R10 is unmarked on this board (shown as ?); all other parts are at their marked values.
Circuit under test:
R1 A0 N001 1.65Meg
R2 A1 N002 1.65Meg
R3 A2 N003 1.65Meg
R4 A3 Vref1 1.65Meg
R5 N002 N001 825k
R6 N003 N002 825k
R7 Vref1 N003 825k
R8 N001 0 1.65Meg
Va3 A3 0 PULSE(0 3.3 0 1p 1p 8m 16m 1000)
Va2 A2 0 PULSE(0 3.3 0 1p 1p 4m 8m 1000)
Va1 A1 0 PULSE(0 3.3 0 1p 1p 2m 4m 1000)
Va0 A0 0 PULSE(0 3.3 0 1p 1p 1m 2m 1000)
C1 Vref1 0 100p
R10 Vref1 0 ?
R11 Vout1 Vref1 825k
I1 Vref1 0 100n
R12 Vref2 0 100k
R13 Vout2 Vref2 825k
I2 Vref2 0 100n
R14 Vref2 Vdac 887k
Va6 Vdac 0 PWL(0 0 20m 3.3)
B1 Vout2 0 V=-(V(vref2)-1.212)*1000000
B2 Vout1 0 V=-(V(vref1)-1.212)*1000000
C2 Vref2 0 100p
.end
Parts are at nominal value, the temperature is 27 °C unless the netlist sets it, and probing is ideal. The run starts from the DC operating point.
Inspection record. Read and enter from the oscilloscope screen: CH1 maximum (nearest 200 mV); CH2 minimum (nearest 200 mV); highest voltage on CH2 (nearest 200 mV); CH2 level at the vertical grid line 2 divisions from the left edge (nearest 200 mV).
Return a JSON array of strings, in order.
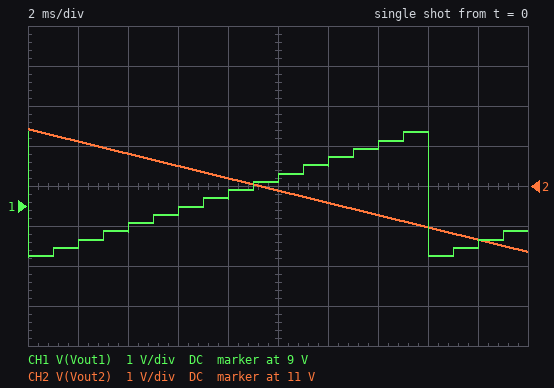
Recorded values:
["10.8 V", "9.4 V", "12.4 V", "11.8 V"]
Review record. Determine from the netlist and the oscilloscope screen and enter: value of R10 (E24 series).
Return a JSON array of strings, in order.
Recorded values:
["120 kΩ"]
